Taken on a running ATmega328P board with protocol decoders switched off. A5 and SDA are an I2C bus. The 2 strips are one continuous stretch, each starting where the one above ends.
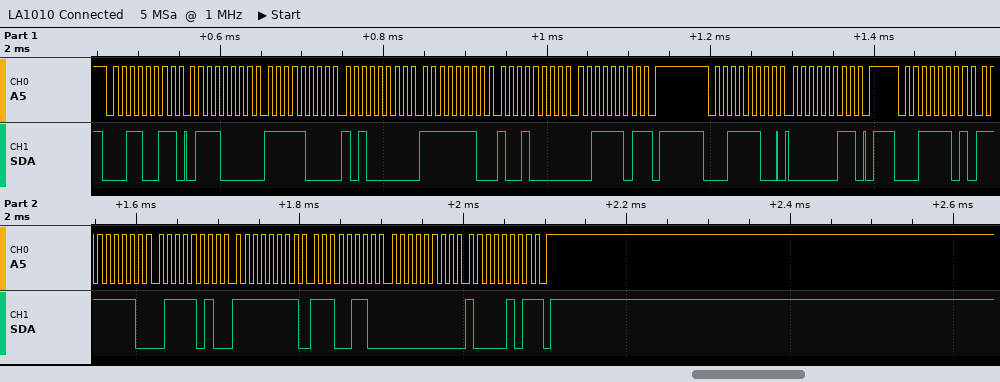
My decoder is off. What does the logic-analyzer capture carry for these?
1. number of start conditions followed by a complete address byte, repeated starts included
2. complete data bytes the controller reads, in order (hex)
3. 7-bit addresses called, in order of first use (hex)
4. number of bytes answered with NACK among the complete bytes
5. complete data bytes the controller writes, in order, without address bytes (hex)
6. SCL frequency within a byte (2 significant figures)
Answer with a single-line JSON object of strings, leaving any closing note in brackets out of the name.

{"number of start conditions followed by a complete address byte, repeated starts included": "3", "complete data bytes the controller reads, in order": "70 F8 A0 FE 90 3D FE 7A FF E6 00 85", "7-bit addresses called, in order of first use": "0x19 0x1E", "number of bytes answered with NACK among the complete bytes": "2", "complete data bytes the controller writes, in order, without address bytes": "03", "SCL frequency within a byte": "100 kHz"}
